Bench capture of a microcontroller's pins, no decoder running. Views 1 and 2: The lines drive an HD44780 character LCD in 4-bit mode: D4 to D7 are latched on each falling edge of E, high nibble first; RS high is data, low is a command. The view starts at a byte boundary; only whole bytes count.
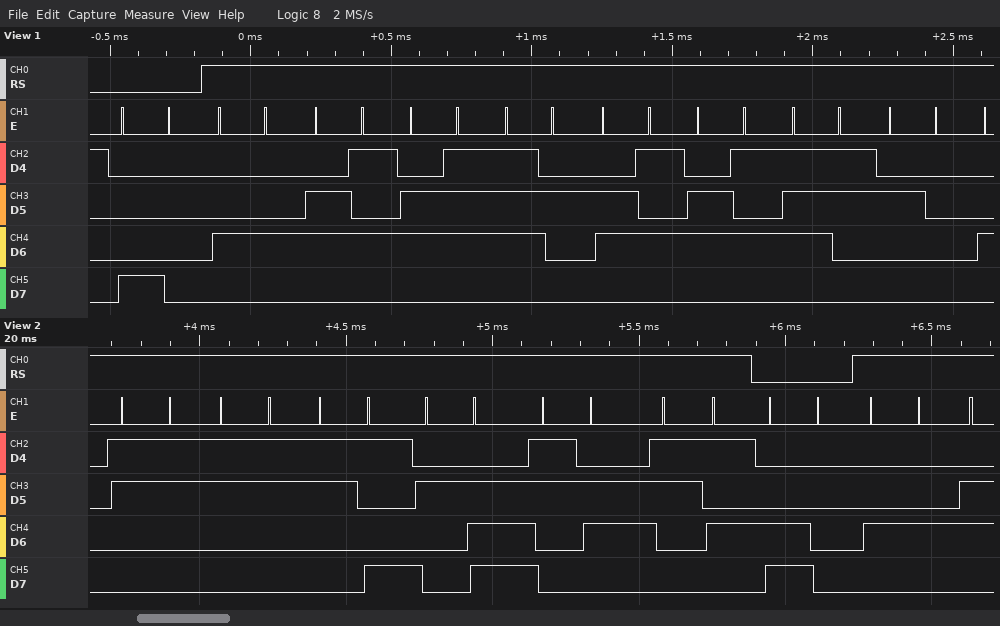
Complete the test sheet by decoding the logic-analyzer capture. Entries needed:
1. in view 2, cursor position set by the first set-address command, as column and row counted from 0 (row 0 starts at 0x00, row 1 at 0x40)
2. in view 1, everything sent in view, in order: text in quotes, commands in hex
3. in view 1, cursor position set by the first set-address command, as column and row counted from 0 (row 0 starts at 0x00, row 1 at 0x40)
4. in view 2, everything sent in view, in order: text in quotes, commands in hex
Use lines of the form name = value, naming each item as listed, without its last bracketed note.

in view 2, cursor position set by the first set-address command, as column and row counted from 0 = column 0, row 1
in view 1, everything sent in view, in order: text in quotes, commands in hex = 0x80 "Degrees "
in view 1, cursor position set by the first set-address command, as column and row counted from 0 = column 0, row 0
in view 2, everything sent in view, in order: text in quotes, commands in hex = "339.65" 0xC0 "D"
